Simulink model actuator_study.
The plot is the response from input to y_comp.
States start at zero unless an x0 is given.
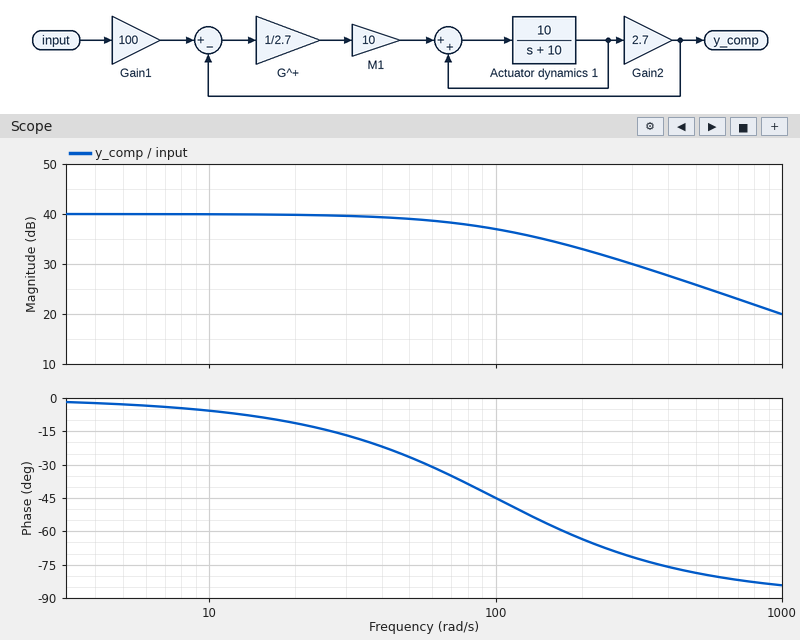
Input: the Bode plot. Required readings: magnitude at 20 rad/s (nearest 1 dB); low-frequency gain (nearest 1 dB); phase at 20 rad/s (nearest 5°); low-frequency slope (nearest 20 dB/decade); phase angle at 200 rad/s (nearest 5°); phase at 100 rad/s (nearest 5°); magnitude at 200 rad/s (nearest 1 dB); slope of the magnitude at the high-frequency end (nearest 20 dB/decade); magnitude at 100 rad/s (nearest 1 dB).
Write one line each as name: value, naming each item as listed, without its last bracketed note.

magnitude at 20 rad/s: 40 dB
low-frequency gain: 40 dB
phase at 20 rad/s: -10°
low-frequency slope: 0 dB/decade
phase angle at 200 rad/s: -65°
phase at 100 rad/s: -45°
magnitude at 200 rad/s: 33 dB
slope of the magnitude at the high-frequency end: -20 dB/decade
magnitude at 100 rad/s: 37 dB
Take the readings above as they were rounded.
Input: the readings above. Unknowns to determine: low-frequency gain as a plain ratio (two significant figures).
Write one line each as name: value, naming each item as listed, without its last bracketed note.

low-frequency gain as a plain ratio: 100
